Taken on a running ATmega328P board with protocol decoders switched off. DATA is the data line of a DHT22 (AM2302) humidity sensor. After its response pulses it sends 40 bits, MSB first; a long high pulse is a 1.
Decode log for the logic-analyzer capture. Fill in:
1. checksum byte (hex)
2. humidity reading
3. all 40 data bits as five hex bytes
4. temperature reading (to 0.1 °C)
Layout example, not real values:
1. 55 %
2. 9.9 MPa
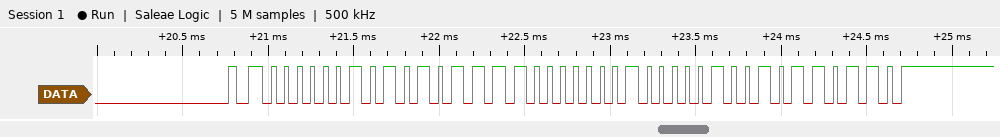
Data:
1. 0xB6
2. 68.7 %
3. 02 AF 01 04 B6
4. 26.0 °C
